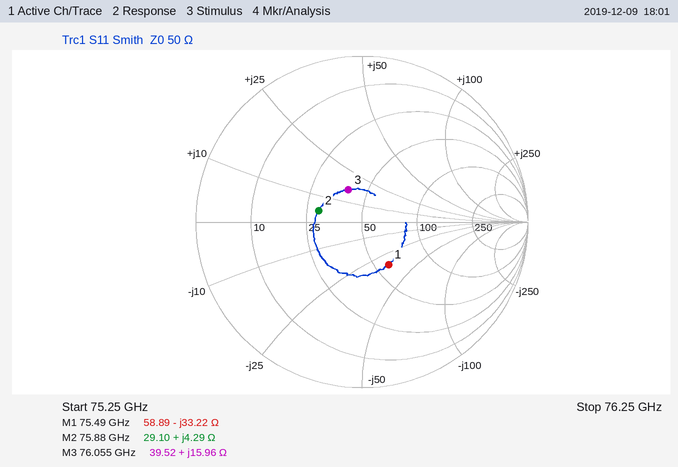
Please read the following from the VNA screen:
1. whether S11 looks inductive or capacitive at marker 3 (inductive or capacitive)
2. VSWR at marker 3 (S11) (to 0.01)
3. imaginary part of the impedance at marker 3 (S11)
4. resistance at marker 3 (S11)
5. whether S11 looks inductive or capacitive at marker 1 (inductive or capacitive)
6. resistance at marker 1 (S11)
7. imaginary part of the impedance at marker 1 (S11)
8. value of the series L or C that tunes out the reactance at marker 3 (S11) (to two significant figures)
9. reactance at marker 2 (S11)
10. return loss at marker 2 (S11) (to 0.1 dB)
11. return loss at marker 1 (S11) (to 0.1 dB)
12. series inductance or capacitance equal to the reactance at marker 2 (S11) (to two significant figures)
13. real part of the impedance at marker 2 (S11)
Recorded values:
inductive
1.53
+15.96 Ω
39.52 Ω
capacitive
58.89 Ω
-33.22 Ω
130 fF
+4.29 Ω
11.4 dB
10.4 dB
9.0 pH
29.10 Ω
